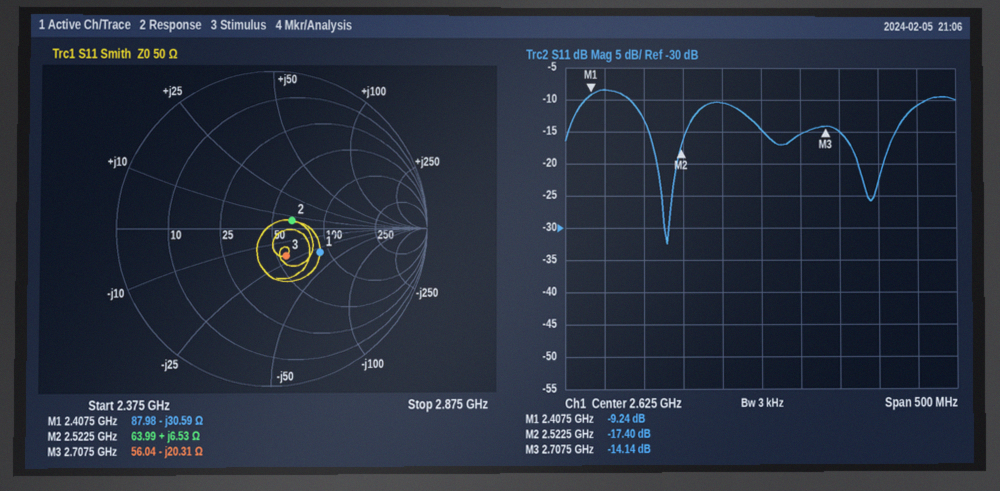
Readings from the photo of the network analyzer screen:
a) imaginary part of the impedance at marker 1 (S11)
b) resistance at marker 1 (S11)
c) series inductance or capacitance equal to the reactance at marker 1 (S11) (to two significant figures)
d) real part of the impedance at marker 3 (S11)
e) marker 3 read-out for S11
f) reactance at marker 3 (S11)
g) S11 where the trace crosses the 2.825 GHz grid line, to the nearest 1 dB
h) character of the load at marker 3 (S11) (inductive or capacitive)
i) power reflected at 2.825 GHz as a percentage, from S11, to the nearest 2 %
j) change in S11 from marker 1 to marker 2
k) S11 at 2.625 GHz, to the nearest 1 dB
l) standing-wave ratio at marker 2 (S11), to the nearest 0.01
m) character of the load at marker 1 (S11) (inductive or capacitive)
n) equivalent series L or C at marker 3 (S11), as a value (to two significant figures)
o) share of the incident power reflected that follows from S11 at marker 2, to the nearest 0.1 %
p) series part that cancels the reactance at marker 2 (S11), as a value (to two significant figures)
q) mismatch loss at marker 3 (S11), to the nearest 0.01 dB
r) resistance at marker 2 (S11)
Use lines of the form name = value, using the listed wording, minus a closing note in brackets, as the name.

imaginary part of the impedance at marker 1 = -30.59 Ω
resistance at marker 1 = 87.98 Ω
series inductance or capacitance equal to the reactance at marker 1 (S11) = 2.2 pF
real part of the impedance at marker 3 = 56.04 Ω
marker 3 read-out for S11 = -14.14 dB
reactance at marker 3 = -20.31 Ω
S11 where the trace crosses the 2.825 GHz grid line, to the nearest 1 dB = -11 dB
character of the load at marker 3 (S11) = capacitive
power reflected at 2.825 GHz as a percentage, from S11, to the nearest 2 % = 8 %
change in S11 from marker 1 to marker 2 = -8.16 dB
S11 at 2.625 GHz, to the nearest 1 dB = -15 dB
standing-wave ratio at marker 2 (S11), to the nearest 0.01 = 1.31
character of the load at marker 1 (S11) = capacitive
equivalent series L or C at marker 3 (S11), as a value = 2.9 pF
share of the incident power reflected that follows from S11 at marker 2, to the nearest 0.1 % = 1.8 %
series part that cancels the reactance at marker 2 (S11), as a value = 9.7 pF
mismatch loss at marker 3 (S11), to the nearest 0.01 dB = 0.17 dB
resistance at marker 2 = 63.99 Ω
